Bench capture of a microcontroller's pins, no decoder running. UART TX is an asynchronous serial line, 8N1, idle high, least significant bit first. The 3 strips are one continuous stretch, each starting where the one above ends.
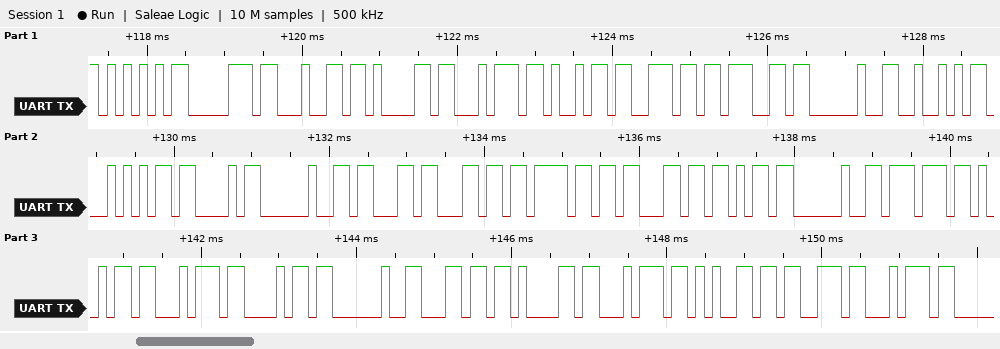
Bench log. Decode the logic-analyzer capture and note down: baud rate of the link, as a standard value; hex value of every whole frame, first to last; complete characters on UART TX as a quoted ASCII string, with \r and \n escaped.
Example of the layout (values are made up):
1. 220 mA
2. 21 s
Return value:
1. 9600 baud
2. 0x55 0x70 0x64 0x61 0x74 0x69 0x6E 0x67 0x20 0x52 0x54 0x43 0x20 0x63 0x6C 0x6F 0x63 0x6B 0x20 0x77 0x69 0x74 0x68 0x20 0x6C 0x61 0x74 0x65 0x73 0x74
3. "Updating RTC clock with latest"
